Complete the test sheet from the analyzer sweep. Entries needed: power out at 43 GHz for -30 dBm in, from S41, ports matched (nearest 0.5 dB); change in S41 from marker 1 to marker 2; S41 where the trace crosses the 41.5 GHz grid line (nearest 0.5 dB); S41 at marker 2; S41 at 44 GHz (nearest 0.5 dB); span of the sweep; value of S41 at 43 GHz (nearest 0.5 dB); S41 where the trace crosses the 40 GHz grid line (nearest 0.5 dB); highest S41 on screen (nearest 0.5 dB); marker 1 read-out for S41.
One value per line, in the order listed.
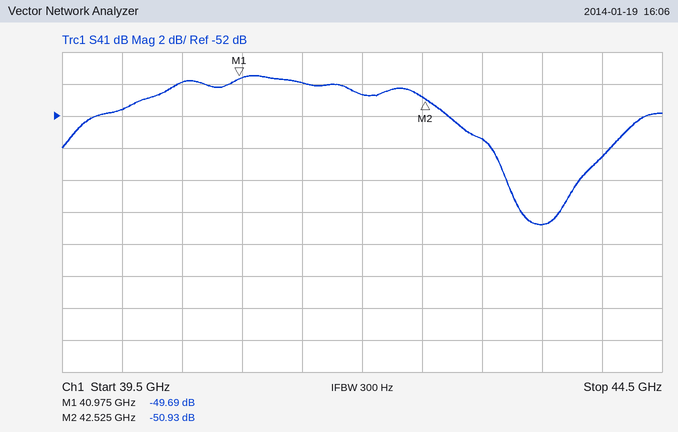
-83.5 dBm
-1.24 dB
-50.0 dB
-50.93 dB
-54.5 dB
5 GHz
-53.5 dB
-51.5 dB
-49.5 dB
-49.69 dB
